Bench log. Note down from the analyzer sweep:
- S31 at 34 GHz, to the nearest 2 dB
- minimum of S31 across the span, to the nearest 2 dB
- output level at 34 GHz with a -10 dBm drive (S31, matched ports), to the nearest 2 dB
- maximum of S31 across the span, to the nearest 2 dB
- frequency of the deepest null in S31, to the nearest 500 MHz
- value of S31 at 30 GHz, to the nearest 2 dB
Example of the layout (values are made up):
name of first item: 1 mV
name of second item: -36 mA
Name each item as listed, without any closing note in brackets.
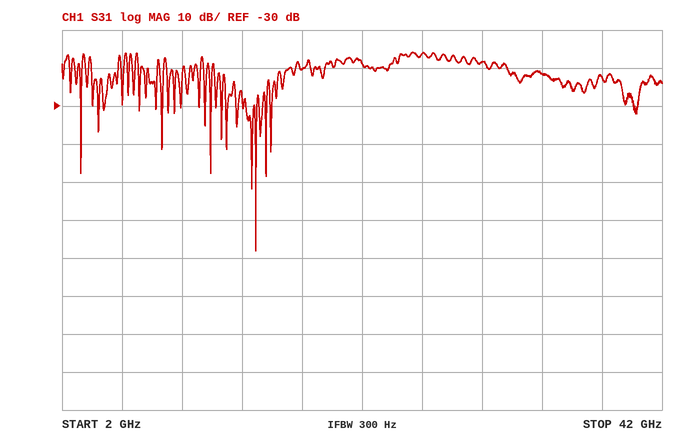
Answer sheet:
S31 at 34 GHz, to the nearest 2 dB: -22 dB
minimum of S31 across the span, to the nearest 2 dB: -68 dB
output level at 34 GHz with a -10 dBm drive (S31, matched ports), to the nearest 2 dB: -32 dBm
maximum of S31 across the span, to the nearest 2 dB: -16 dB
frequency of the deepest null in S31, to the nearest 500 MHz: 15.0 GHz
value of S31 at 30 GHz, to the nearest 2 dB: -18 dB
